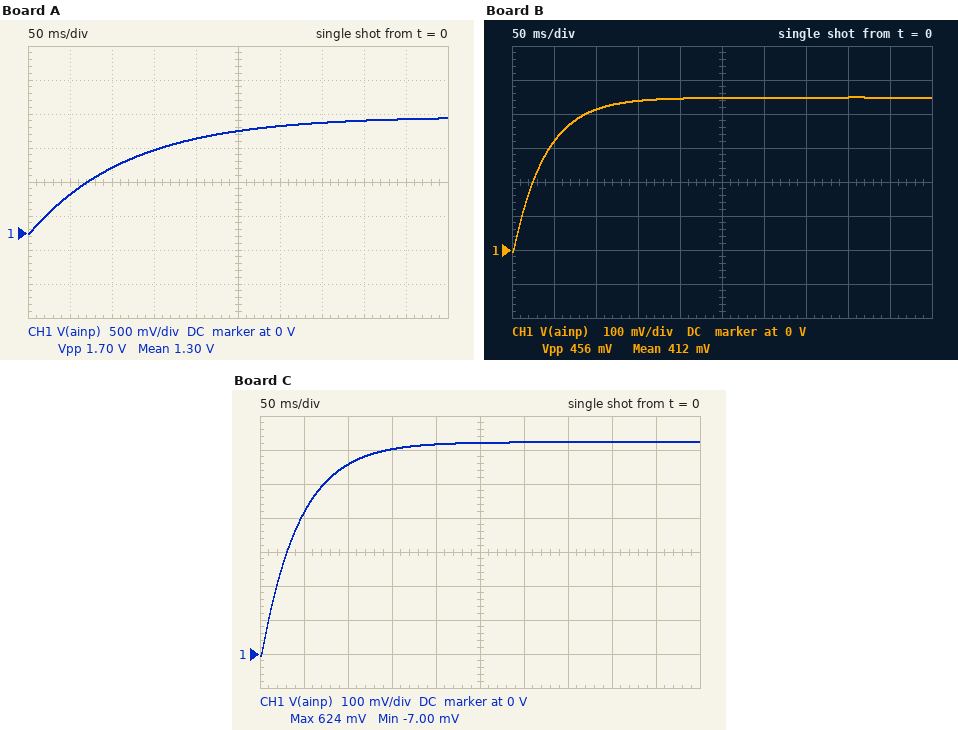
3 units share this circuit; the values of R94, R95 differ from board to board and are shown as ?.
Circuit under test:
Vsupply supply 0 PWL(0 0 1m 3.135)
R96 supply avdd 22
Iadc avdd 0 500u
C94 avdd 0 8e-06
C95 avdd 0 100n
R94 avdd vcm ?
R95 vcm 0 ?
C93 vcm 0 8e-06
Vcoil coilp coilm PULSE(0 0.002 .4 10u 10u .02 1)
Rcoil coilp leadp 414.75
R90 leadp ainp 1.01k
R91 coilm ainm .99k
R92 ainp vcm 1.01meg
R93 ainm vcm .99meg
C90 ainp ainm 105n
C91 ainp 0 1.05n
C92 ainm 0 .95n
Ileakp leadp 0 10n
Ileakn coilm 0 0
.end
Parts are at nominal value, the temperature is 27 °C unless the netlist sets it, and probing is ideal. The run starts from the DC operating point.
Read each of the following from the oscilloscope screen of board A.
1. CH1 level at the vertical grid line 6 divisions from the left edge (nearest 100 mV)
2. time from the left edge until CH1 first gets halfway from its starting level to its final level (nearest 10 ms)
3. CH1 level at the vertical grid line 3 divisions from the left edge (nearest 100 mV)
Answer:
1.6 V
80 ms
1.2 V
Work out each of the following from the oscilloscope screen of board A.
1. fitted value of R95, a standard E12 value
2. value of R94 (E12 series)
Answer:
33 kΩ
27 kΩ
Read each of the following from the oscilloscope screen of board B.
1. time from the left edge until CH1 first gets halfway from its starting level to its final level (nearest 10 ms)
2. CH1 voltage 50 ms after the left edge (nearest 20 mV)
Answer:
30 ms
320 mV
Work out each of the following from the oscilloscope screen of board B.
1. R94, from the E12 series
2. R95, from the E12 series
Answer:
33 kΩ
5.6 kΩ
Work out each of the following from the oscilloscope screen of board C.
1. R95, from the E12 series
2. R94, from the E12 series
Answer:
6.8 kΩ
27 kΩ
